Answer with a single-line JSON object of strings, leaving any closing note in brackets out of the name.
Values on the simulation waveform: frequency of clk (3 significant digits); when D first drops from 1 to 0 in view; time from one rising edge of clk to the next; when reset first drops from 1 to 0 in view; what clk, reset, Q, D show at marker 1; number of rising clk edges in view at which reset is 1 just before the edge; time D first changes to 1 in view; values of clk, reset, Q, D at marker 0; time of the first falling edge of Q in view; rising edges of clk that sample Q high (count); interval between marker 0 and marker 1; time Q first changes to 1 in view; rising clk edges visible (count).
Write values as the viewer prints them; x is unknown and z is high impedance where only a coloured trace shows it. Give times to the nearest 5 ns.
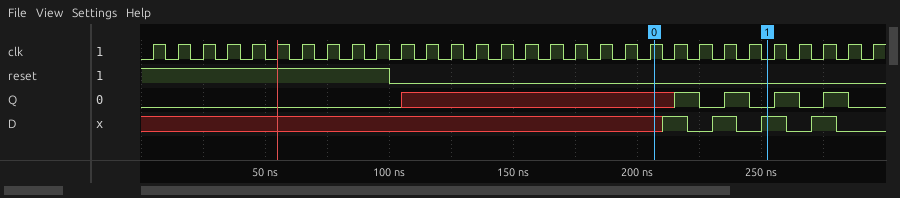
{"frequency of clk": "100 MHz", "when D first drops from 1 to 0 in view": "220 ns", "time from one rising edge of clk to the next": "10 ns", "when reset first drops from 1 to 0 in view": "100 ns", "what clk, reset, Q, D show at marker 1": "clk=0, reset=0, Q=0, D=1", "number of rising clk edges in view at which reset is 1 just before the edge": "10", "time D first changes to 1 in view": "210 ns", "values of clk, reset, Q, D at marker 0": "clk=1, reset=0, Q=x, D=x", "time of the first falling edge of Q in view": "225 ns", "rising edges of clk that sample Q high": "4", "interval between marker 0 and marker 1": "45 ns", "time Q first changes to 1 in view": "215 ns", "rising clk edges visible": "30"}
